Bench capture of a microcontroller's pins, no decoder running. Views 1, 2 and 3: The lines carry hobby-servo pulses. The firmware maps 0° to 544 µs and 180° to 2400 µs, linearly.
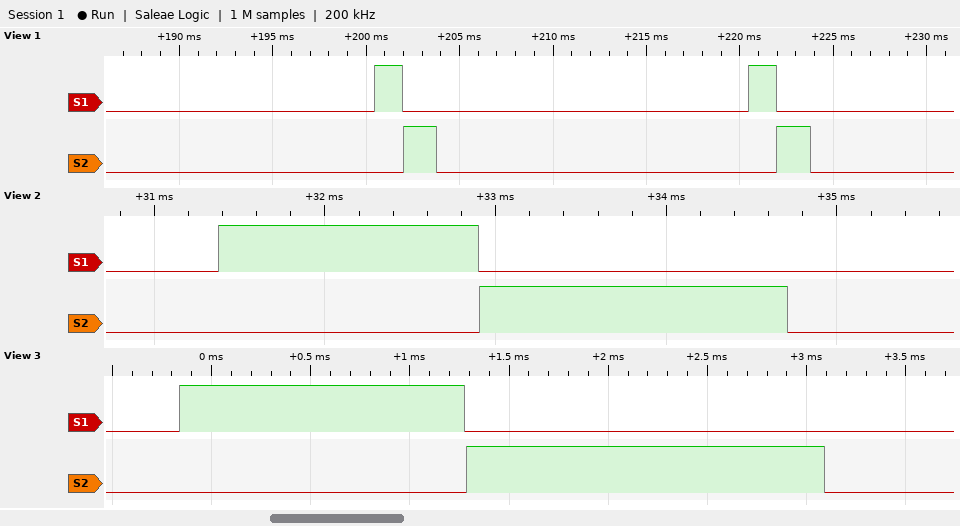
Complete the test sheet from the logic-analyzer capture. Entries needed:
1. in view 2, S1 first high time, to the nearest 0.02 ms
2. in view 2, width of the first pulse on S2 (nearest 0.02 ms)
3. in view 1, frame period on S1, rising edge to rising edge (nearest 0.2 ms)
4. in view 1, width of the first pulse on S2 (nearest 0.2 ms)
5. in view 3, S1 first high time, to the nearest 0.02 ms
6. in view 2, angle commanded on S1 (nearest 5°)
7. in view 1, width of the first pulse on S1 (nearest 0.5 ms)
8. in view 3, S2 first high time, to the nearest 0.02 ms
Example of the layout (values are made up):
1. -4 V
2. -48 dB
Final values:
1. 1.52 ms
2. 1.80 ms
3. 20.0 ms
4. 1.8 ms
5. 1.44 ms
6. 95°
7. 1.5 ms
8. 1.80 ms
